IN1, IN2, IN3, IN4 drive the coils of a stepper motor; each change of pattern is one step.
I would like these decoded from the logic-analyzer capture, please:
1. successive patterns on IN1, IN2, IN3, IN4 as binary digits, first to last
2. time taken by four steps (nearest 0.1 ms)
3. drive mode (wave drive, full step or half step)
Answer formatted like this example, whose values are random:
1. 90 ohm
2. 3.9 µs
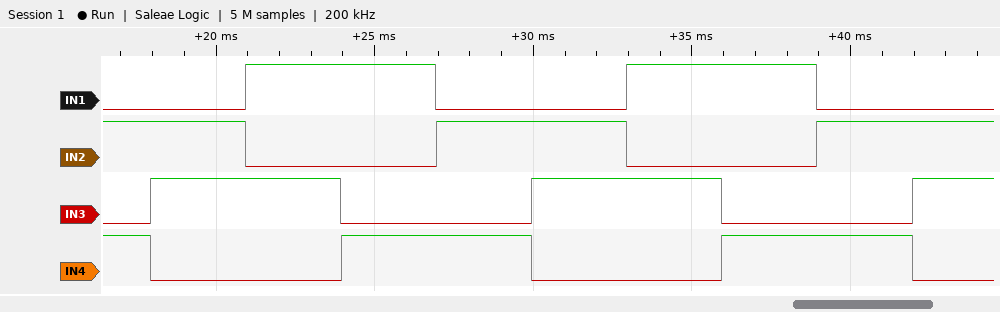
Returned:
1. 0101 0110 1010 1001 0101 0110 1010 1001 0101 0110
2. 12.0 ms
3. full step
